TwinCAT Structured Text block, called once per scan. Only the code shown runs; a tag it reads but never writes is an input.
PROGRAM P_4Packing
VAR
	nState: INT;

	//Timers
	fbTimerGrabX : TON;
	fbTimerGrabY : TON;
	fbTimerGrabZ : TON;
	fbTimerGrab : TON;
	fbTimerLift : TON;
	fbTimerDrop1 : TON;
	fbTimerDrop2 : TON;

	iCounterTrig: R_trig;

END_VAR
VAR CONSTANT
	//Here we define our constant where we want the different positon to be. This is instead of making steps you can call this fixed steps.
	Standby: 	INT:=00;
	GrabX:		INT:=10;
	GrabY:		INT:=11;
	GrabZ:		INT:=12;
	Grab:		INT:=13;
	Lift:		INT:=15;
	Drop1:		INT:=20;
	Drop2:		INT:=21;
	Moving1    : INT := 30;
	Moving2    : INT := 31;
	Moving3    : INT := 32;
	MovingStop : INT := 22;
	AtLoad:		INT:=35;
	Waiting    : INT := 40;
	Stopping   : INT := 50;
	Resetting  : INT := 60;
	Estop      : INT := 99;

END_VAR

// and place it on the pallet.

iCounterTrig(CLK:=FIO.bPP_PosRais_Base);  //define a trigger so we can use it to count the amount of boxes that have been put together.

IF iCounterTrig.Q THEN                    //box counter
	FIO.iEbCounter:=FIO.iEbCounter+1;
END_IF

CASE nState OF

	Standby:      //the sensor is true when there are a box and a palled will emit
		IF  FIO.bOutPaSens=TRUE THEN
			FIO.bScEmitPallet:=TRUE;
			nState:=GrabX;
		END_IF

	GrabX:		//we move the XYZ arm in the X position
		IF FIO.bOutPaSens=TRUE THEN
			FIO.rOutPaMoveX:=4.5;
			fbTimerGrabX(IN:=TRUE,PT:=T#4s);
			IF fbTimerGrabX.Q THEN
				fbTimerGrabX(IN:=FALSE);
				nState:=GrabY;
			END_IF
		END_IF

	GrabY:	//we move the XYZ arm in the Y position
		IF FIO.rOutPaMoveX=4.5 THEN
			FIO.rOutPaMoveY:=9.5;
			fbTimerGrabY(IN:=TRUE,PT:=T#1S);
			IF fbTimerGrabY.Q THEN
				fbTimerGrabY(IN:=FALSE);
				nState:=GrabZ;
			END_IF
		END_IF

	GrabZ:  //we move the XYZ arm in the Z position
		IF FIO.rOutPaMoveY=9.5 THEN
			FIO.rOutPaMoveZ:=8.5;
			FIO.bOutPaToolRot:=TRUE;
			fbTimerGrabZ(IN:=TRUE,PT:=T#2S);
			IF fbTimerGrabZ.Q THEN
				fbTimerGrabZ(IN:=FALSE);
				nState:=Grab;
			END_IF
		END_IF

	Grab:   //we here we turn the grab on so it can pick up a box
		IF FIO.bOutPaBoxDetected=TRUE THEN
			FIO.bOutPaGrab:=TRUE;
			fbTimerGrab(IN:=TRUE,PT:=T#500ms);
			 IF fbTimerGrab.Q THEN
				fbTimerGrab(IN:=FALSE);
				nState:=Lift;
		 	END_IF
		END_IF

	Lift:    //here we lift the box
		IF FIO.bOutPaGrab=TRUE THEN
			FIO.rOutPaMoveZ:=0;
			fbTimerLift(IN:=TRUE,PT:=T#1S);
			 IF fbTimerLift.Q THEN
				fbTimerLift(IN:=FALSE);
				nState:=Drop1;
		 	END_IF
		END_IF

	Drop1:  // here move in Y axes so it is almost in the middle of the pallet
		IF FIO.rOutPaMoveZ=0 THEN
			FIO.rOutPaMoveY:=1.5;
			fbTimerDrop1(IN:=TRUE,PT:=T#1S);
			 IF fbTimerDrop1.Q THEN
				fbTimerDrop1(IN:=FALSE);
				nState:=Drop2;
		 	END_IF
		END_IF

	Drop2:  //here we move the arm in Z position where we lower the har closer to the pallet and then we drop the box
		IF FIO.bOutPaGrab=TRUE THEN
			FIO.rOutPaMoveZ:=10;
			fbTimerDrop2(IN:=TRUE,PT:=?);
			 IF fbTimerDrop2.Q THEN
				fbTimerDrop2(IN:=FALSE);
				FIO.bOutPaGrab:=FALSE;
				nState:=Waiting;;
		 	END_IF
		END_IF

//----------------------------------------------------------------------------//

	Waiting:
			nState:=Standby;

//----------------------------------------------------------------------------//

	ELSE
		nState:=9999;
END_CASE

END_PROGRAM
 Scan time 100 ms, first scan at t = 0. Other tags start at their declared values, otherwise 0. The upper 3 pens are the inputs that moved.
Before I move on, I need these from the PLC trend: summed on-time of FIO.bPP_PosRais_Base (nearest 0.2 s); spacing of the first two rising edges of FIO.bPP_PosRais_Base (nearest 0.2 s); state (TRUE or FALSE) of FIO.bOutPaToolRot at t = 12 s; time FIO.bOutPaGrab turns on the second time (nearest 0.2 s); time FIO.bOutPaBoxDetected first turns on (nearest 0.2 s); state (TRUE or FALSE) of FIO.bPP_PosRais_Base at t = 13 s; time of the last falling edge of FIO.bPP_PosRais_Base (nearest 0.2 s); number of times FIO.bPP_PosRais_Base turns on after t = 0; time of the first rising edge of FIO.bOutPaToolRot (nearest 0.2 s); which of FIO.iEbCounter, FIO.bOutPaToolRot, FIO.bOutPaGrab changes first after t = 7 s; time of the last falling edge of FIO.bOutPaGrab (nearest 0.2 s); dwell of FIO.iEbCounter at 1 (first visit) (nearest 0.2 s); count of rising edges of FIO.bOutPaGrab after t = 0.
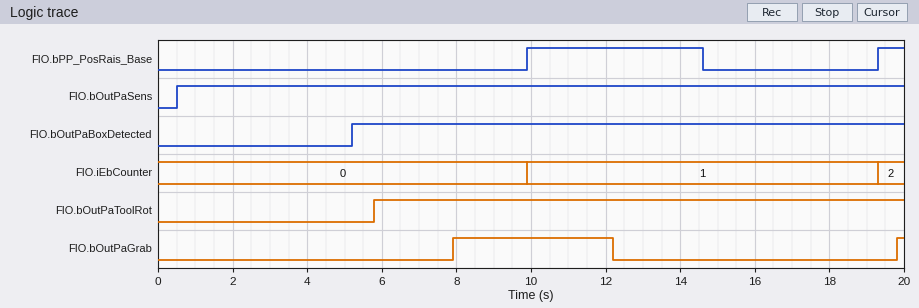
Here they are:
5.4 s
9.4 s
TRUE
19.8 s
5.2 s
TRUE
14.6 s
2
5.8 s
FIO.bOutPaGrab
12.2 s
9.4 s
2
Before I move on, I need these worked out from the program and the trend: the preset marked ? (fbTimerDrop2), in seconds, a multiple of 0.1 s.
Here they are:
1.5 s
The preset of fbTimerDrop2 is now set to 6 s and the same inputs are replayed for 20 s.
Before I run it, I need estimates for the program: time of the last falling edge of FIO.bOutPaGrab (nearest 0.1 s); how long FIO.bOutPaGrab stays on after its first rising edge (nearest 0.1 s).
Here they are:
16.7 s
8.8 s
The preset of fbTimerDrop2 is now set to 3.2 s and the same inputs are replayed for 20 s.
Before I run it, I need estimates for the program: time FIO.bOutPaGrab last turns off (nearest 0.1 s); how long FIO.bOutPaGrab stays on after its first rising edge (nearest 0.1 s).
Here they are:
13.9 s
6.0 s
